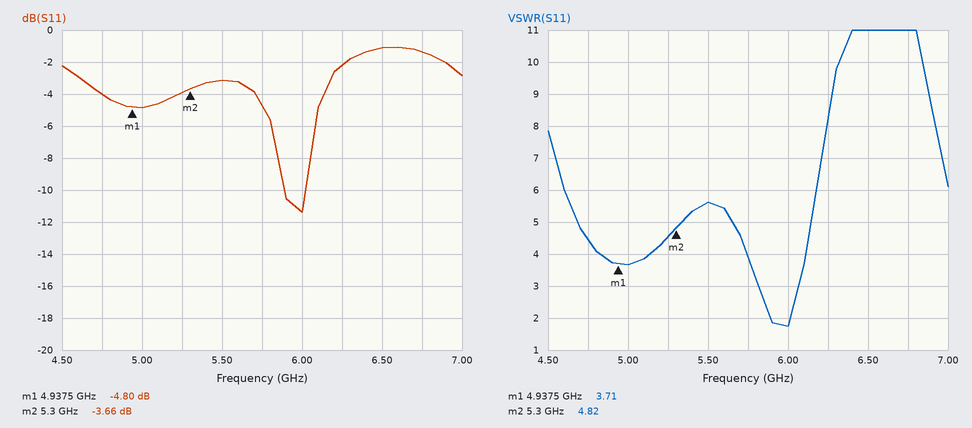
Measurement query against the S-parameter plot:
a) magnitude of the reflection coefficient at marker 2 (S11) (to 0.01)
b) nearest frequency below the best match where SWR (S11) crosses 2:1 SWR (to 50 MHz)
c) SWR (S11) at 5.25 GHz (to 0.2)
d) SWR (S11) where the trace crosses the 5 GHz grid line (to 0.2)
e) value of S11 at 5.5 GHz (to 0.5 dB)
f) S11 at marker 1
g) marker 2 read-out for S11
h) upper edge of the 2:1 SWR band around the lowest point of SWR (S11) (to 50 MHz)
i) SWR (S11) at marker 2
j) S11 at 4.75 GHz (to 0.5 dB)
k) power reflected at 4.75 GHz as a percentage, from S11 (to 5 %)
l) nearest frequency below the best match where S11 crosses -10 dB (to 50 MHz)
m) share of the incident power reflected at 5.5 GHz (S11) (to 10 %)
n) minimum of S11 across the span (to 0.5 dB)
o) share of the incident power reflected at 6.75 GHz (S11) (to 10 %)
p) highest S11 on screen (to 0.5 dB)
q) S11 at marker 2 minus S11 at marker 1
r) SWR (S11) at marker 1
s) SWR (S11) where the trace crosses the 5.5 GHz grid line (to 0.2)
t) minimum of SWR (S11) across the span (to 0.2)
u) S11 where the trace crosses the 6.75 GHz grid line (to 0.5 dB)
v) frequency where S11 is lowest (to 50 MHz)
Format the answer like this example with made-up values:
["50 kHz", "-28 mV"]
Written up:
["0.66", "5.90 GHz", "4.6", "3.6", "-3.0 dB", "-4.80 dB", "-3.66 dB", "6.00 GHz", "4.82", "-4.0 dB", "40 %", "5.90 GHz", "50 %", "-11.5 dB", "70 %", "-1.0 dB", "1.14 dB", "3.71", "5.6", "1.8", "-1.5 dB", "6.00 GHz"]
